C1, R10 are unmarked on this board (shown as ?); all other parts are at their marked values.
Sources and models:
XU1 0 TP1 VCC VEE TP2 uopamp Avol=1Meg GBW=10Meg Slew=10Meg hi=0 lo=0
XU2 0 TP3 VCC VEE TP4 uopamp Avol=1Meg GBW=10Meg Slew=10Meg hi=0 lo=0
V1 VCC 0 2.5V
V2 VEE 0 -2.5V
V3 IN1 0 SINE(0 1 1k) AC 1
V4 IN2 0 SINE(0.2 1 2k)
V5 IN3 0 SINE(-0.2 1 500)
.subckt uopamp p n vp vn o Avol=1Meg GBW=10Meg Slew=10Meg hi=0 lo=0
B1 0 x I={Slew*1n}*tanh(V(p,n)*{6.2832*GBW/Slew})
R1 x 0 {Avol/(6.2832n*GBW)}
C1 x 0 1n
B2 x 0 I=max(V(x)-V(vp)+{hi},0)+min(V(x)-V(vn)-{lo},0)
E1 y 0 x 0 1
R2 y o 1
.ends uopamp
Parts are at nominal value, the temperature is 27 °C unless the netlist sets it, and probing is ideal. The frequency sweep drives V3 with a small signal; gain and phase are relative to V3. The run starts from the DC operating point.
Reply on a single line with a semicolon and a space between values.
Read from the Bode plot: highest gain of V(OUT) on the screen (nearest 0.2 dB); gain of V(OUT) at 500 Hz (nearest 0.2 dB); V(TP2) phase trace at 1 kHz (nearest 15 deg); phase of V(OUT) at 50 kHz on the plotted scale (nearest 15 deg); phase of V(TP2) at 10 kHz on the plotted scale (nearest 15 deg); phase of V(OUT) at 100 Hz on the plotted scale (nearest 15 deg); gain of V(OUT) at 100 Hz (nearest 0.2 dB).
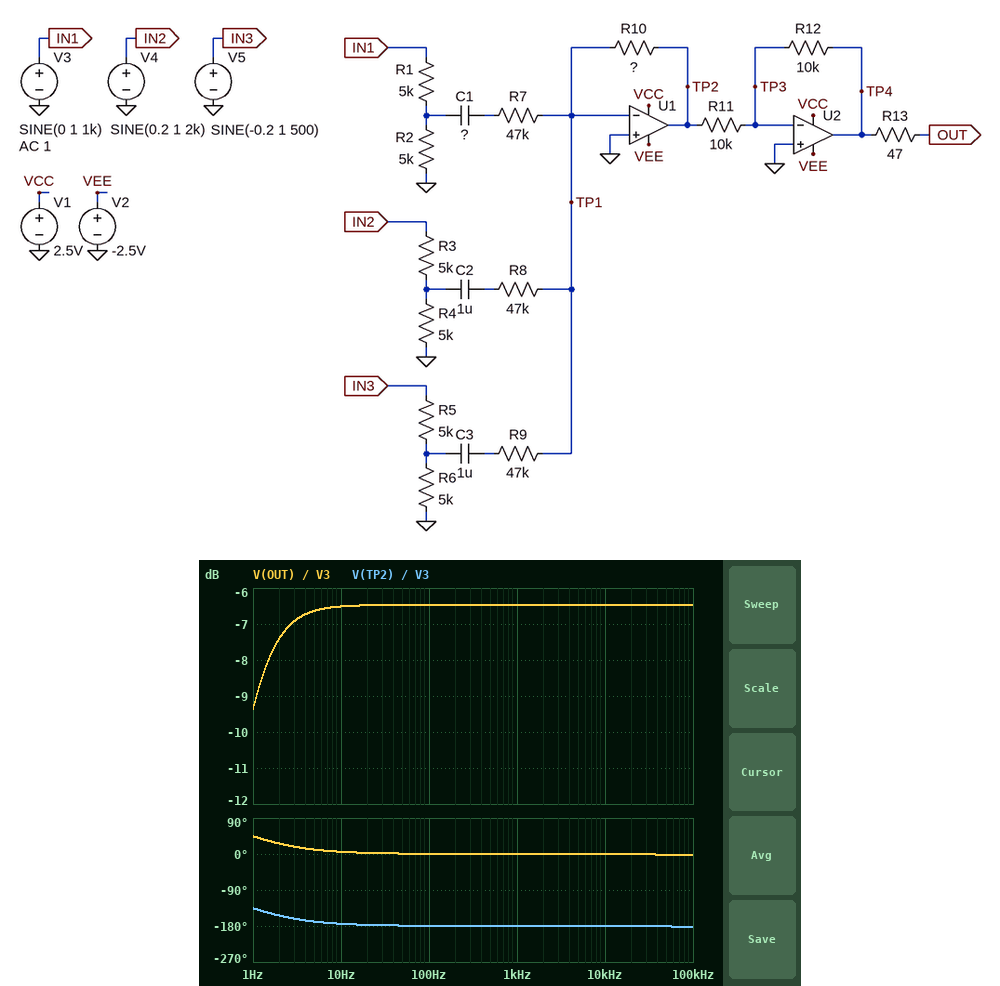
-6.4 dB; -6.4 dB; -180 deg; 0 deg; -180 deg; 0 deg; -6.4 dB
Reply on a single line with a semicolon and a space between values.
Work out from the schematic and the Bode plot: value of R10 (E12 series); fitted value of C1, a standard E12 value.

47 kΩ; 3.3 µF
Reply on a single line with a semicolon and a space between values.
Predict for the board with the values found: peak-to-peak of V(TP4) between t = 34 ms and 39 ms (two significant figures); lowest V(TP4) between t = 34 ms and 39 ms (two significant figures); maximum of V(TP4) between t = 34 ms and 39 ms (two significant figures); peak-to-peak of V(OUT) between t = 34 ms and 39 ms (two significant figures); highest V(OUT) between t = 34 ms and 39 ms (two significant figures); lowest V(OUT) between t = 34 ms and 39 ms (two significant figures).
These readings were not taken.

2.1 V; -1.1 V; 1.1 V; 2.1 V; 1.1 V; -1.1 V
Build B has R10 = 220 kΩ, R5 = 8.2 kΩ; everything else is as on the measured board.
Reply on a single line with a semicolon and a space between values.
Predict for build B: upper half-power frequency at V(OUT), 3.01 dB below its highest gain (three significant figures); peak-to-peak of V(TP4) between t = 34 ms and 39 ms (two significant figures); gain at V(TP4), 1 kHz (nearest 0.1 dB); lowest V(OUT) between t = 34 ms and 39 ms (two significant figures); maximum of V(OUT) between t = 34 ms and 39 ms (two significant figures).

687 kHz; 5.0 V; 6.9 dB; -2.5 V; 2.5 V
